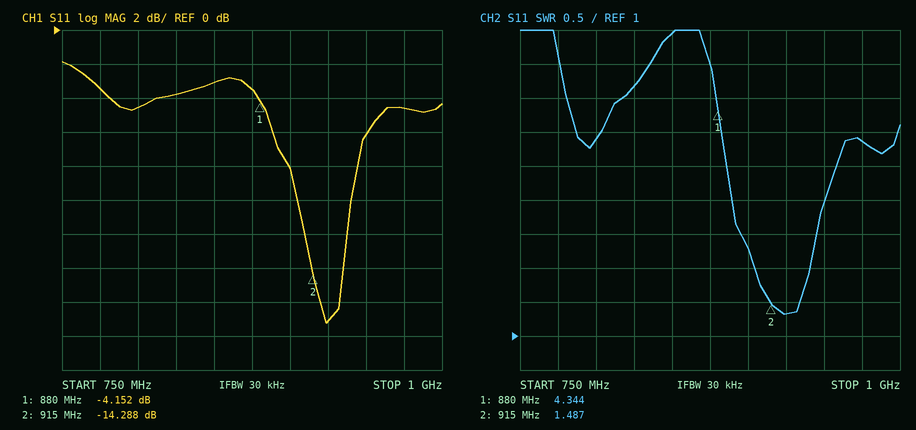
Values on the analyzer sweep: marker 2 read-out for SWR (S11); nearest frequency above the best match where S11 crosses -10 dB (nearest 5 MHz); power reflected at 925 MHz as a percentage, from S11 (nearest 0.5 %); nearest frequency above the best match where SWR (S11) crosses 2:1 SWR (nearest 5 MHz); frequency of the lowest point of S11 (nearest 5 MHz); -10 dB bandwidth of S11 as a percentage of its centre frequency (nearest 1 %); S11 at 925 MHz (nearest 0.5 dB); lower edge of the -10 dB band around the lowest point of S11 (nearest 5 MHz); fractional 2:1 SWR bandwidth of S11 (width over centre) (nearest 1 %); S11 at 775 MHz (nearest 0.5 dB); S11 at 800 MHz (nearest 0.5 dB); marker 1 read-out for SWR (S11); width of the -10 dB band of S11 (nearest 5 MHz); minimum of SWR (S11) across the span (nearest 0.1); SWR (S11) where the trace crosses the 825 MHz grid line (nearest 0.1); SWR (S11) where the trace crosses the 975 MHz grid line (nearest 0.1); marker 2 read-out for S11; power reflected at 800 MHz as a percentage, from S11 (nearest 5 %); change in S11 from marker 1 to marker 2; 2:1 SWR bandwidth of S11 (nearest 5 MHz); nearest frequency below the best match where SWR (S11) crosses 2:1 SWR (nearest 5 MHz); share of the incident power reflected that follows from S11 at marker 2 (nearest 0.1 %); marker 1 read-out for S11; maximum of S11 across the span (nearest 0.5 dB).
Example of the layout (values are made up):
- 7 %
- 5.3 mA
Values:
- 1.487
- 940 MHz
- 2.0 %
- 940 MHz
- 925 MHz
- 4 %
- -17.0 dB
- 905 MHz
- 4 %
- -3.5 dB
- -4.5 dB
- 4.344
- 35 MHz
- 1.3
- 4.7
- 3.9
- -14.288 dB
- 35 %
- -10.136 dB
- 35 MHz
- 905 MHz
- 3.7 %
- -4.152 dB
- -2.0 dB
